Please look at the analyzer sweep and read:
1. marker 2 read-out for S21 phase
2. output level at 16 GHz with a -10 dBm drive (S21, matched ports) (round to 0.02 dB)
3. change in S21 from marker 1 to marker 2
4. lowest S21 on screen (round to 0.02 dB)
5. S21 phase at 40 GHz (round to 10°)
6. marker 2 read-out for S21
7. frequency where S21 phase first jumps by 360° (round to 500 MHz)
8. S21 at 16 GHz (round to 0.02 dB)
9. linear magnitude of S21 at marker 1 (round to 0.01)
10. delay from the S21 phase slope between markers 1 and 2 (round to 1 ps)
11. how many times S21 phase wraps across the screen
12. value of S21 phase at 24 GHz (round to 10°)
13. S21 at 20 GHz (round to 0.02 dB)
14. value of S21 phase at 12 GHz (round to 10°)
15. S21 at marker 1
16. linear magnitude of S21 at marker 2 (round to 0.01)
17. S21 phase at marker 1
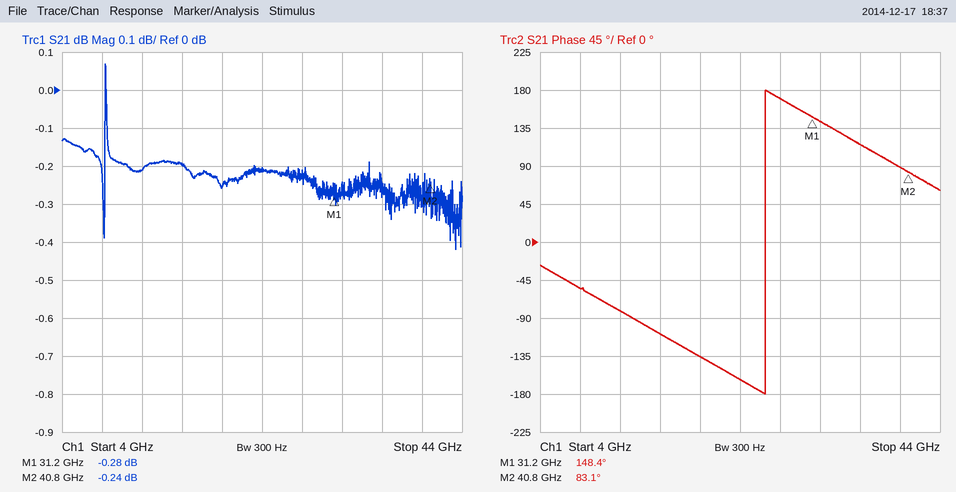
83.1°
-10.20 dBm
0.04 dB
-0.42 dB
90°
-0.24 dB
26.5 GHz
-0.20 dB
0.97
19 ps
1
-160°
-0.26 dB
-80°
-0.28 dB
0.97
148.4°
